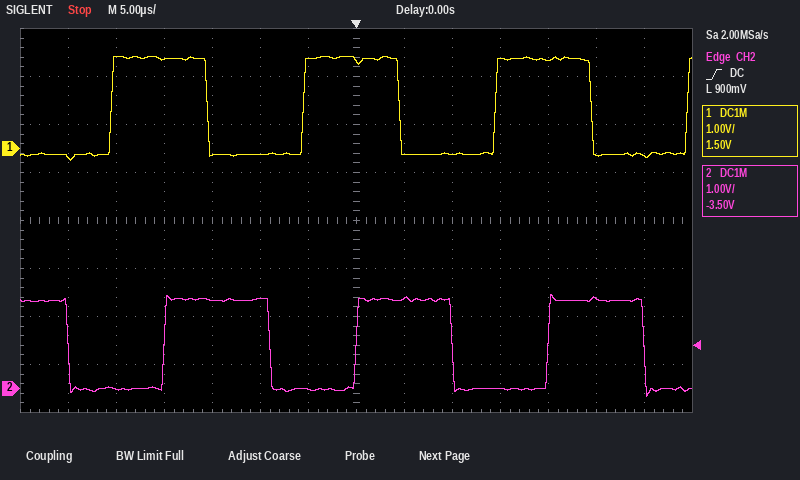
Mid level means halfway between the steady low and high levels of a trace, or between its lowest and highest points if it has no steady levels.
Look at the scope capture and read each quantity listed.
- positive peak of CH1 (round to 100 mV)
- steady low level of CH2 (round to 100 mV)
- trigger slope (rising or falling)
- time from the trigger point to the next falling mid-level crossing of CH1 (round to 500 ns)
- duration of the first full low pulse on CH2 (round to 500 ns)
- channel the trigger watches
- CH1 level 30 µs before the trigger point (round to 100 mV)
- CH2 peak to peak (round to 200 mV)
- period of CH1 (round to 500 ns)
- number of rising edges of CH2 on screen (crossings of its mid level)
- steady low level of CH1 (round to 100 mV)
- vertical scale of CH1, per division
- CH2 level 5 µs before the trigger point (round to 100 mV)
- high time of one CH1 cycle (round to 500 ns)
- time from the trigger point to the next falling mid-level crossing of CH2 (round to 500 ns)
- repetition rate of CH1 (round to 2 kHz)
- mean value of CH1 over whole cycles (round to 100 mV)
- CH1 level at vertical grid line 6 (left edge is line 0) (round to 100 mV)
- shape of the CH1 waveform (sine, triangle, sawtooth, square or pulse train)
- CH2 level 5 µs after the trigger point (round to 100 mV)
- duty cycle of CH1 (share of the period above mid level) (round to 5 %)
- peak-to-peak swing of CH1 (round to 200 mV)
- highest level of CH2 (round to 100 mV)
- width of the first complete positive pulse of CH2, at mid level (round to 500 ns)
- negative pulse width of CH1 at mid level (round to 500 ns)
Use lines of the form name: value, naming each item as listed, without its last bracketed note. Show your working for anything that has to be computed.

positive peak of CH1: 1.9 V
steady low level of CH2: 0.0 V
trigger slope: rising
time from the trigger point to the next falling mid-level crossing of CH1: 4.5 µs
duration of the first full low pulse on CH2: 10.0 µs
channel the trigger watches: CH2
CH1 level 30 µs before the trigger point: -200 mV
CH2 peak to peak: 2.2 V
period of CH1: 20.0 µs
number of rising edges of CH2 on screen: 3
steady low level of CH1: -100 mV
vertical scale of CH1, per division: 1 V
CH2 level 5 µs before the trigger point: 0.0 V
high time of one CH1 cycle: 10.0 µs
time from the trigger point to the next falling mid-level crossing of CH2: 10.0 µs
repetition rate of CH1: 1 / 20.0 µs ≈ 50 kHz
mean value of CH1 over whole cycles: -100 mV + 0.5 × (1.9 V − (-100 mV)) ≈ 900 mV
CH1 level at vertical grid line 6 (left edge is line 0): 1.9 V
shape of the CH1 waveform: square
CH2 level 5 µs after the trigger point: 1.9 V
duty cycle of CH1 (share of the period above mid level): 10.0 µs / 20.0 µs ≈ 50 %
peak-to-peak swing of CH1: 2.2 V
highest level of CH2: 2.0 V
width of the first complete positive pulse of CH2, at mid level: 11.0 µs
negative pulse width of CH1 at mid level: 10.0 µs
